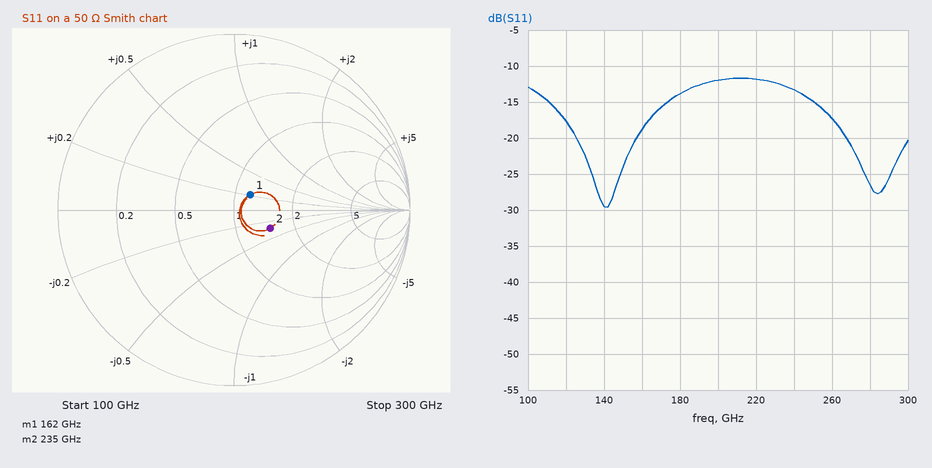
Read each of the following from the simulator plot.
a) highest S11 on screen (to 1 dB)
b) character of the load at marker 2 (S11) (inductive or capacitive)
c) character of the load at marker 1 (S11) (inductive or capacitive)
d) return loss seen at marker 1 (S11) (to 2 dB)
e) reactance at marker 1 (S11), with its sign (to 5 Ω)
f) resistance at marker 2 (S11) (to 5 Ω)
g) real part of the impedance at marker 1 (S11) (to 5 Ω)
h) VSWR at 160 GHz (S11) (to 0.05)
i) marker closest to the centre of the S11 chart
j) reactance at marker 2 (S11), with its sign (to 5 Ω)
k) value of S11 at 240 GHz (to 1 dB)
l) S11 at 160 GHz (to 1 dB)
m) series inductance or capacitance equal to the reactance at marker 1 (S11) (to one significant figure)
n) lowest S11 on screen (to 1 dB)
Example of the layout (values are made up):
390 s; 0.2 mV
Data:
-12 dB; capacitive; inductive; 18 dB; +10 Ω; 75 Ω; 60 Ω; 1.25; marker 1; -15 Ω; -13 dB; -19 dB; 10 pH; -30 dB
